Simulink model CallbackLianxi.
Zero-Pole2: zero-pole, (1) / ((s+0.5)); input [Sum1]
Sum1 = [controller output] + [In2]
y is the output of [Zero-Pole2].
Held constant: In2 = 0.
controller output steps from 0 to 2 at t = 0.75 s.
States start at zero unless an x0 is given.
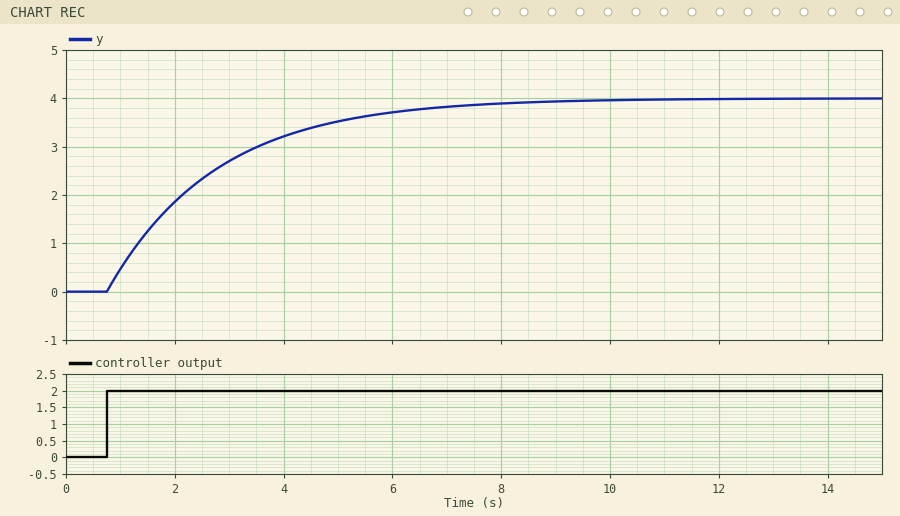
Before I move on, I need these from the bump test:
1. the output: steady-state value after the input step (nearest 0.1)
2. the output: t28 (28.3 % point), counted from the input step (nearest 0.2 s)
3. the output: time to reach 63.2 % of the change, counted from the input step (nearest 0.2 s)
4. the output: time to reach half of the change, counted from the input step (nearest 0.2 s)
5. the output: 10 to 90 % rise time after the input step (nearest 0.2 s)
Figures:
4.0
0.6 s
2.0 s
1.4 s
4.4 s
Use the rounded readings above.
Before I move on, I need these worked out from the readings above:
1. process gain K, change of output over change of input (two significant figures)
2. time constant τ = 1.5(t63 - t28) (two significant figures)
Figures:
2.0
2.1 s
